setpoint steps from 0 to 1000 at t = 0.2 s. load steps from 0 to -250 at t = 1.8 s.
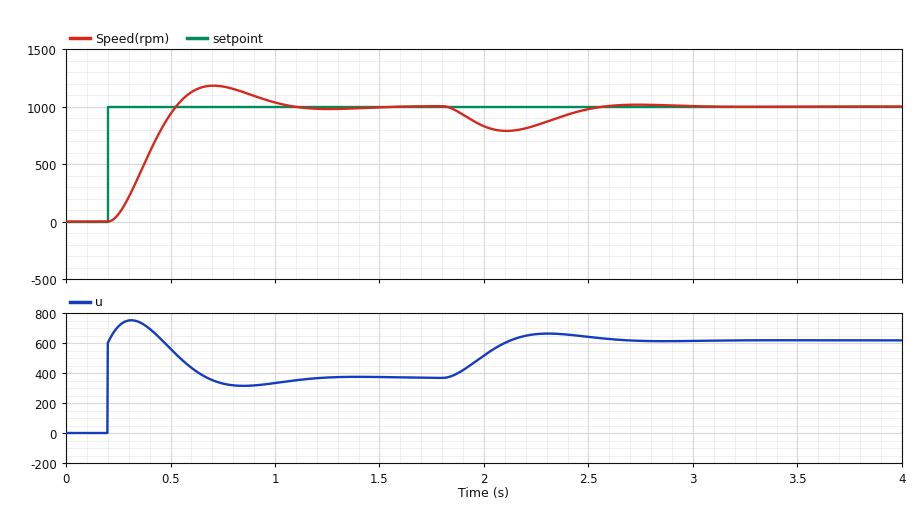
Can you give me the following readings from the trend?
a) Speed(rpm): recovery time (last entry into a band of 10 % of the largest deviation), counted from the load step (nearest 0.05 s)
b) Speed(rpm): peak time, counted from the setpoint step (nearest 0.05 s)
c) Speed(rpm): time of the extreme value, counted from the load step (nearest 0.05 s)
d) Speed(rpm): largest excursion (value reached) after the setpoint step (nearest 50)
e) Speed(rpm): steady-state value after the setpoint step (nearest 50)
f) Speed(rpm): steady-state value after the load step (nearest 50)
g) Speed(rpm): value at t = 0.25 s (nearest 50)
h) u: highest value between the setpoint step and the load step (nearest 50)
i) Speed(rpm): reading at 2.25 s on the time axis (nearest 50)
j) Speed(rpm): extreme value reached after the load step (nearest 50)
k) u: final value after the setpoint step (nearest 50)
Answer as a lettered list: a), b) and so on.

a) 0.70 s
b) 0.50 s
c) 0.30 s
d) 1200
e) 1000
f) 1000
g) 50
h) 750
i) 850
j) 800
k) 350
